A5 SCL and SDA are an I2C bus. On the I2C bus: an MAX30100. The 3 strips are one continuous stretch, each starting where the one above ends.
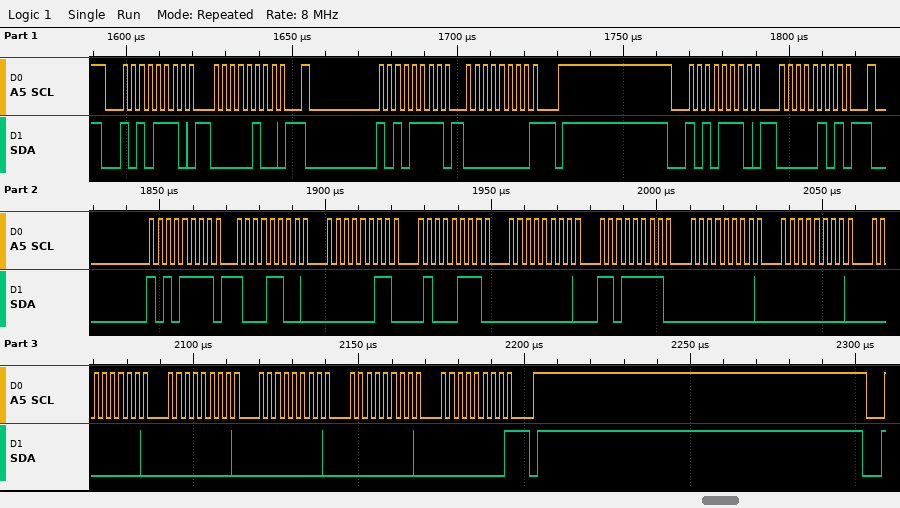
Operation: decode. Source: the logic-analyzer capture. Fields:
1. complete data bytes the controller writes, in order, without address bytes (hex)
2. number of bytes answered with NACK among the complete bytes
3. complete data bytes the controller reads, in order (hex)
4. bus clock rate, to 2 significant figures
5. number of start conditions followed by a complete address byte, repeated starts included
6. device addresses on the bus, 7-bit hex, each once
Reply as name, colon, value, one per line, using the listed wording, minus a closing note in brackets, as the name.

complete data bytes the controller writes, in order, without address bytes: 04 05
number of bytes answered with NACK among the complete bytes: 2
complete data bytes the controller reads, in order: 00 8C 03 47 00 DF 00 00 00 00 00 00 00
bus clock rate, to 2 significant figures: 400 kHz
number of start conditions followed by a complete address byte, repeated starts included: 4
device addresses on the bus, 7-bit hex, each once: 0x57
